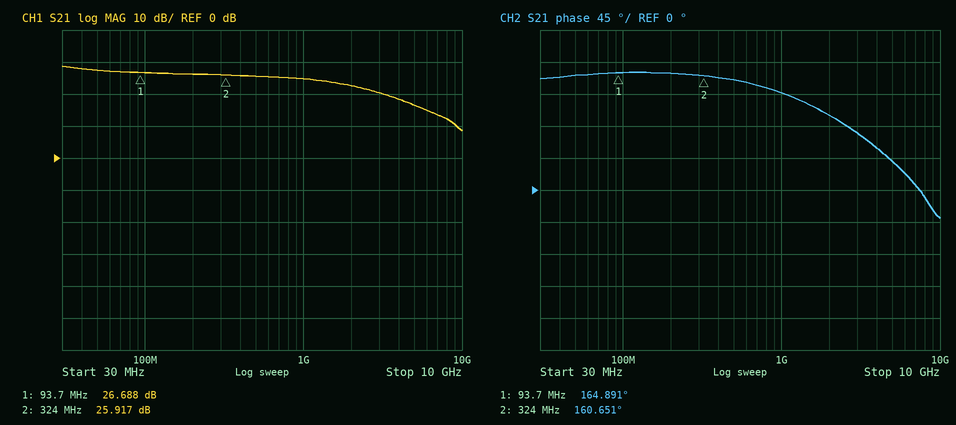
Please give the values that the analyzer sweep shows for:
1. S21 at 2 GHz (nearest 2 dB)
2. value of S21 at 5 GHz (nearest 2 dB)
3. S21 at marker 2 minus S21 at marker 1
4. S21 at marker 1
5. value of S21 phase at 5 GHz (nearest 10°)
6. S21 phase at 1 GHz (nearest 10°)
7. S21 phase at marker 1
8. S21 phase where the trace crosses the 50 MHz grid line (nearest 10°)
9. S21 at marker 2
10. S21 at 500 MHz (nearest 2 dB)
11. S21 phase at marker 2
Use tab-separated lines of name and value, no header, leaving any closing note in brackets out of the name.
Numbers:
S21 at 2 GHz	22 dB
value of S21 at 5 GHz	16 dB
S21 at marker 2 minus S21 at marker 1	-0.771 dB
S21 at marker 1	26.688 dB
value of S21 phase at 5 GHz	40°
S21 phase at 1 GHz	140°
S21 phase at marker 1	164.891°
S21 phase where the trace crosses the 50 MHz grid line	160°
S21 at marker 2	25.917 dB
S21 at 500 MHz	26 dB
S21 phase at marker 2	160.651°
